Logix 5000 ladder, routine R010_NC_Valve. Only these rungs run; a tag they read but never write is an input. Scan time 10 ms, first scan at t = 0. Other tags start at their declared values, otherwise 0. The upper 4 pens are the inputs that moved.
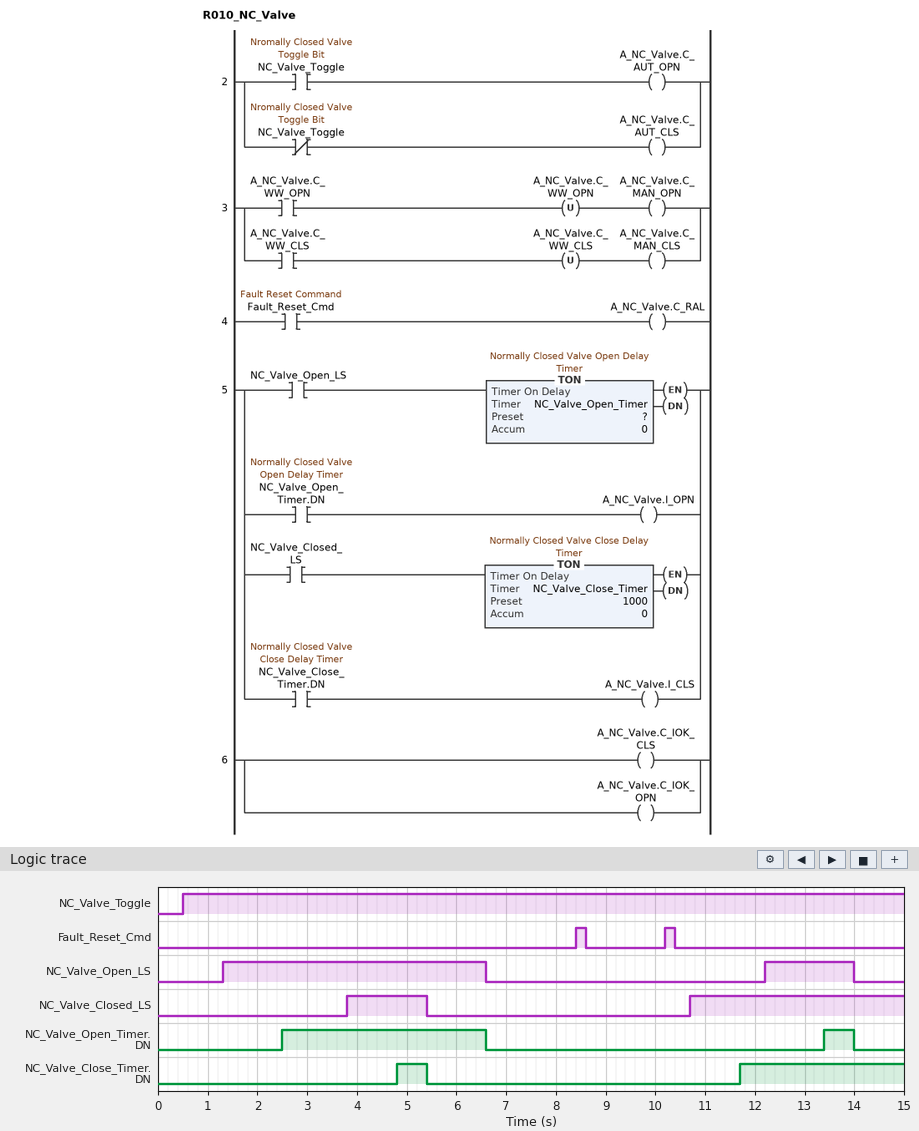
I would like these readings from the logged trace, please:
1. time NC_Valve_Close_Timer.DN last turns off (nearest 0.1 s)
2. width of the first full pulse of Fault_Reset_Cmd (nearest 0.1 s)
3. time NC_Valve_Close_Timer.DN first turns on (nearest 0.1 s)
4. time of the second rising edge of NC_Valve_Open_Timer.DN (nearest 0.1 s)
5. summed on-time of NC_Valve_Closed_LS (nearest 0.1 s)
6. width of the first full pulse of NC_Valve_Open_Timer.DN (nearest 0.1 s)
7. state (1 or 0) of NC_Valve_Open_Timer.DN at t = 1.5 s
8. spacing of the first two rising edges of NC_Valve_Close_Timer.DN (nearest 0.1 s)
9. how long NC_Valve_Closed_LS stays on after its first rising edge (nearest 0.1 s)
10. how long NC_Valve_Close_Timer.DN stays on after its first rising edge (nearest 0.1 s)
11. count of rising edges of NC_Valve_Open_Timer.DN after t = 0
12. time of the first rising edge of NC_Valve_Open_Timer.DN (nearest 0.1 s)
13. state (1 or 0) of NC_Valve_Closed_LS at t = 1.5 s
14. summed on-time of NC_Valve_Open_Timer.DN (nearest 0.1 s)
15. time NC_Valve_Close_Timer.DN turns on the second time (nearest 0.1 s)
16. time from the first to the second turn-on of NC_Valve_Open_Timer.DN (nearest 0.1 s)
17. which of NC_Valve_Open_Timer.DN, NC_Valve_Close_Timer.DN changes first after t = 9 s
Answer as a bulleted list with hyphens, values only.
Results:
- 5.4 s
- 0.2 s
- 4.8 s
- 13.4 s
- 5.9 s
- 4.1 s
- 0
- 6.9 s
- 1.6 s
- 0.6 s
- 2
- 2.5 s
- 0
- 4.7 s
- 11.7 s
- 10.9 s
- NC_Valve_Close_Timer.DN
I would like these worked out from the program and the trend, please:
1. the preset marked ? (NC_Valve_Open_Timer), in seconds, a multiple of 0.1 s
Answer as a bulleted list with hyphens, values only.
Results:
- 1.2 s
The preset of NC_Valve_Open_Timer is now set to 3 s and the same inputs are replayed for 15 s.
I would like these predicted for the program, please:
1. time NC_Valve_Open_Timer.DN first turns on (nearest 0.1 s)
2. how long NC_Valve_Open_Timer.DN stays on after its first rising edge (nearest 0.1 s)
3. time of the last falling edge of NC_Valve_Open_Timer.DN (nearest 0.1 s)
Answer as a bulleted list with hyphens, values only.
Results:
- 4.3 s
- 2.3 s
- 6.6 s
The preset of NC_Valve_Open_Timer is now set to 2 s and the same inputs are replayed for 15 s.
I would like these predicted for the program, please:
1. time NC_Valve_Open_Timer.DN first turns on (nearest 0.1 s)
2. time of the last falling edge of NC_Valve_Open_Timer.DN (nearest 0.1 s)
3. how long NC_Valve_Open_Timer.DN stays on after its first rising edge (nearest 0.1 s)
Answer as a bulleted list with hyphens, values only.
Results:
- 3.3 s
- 6.6 s
- 3.3 s
